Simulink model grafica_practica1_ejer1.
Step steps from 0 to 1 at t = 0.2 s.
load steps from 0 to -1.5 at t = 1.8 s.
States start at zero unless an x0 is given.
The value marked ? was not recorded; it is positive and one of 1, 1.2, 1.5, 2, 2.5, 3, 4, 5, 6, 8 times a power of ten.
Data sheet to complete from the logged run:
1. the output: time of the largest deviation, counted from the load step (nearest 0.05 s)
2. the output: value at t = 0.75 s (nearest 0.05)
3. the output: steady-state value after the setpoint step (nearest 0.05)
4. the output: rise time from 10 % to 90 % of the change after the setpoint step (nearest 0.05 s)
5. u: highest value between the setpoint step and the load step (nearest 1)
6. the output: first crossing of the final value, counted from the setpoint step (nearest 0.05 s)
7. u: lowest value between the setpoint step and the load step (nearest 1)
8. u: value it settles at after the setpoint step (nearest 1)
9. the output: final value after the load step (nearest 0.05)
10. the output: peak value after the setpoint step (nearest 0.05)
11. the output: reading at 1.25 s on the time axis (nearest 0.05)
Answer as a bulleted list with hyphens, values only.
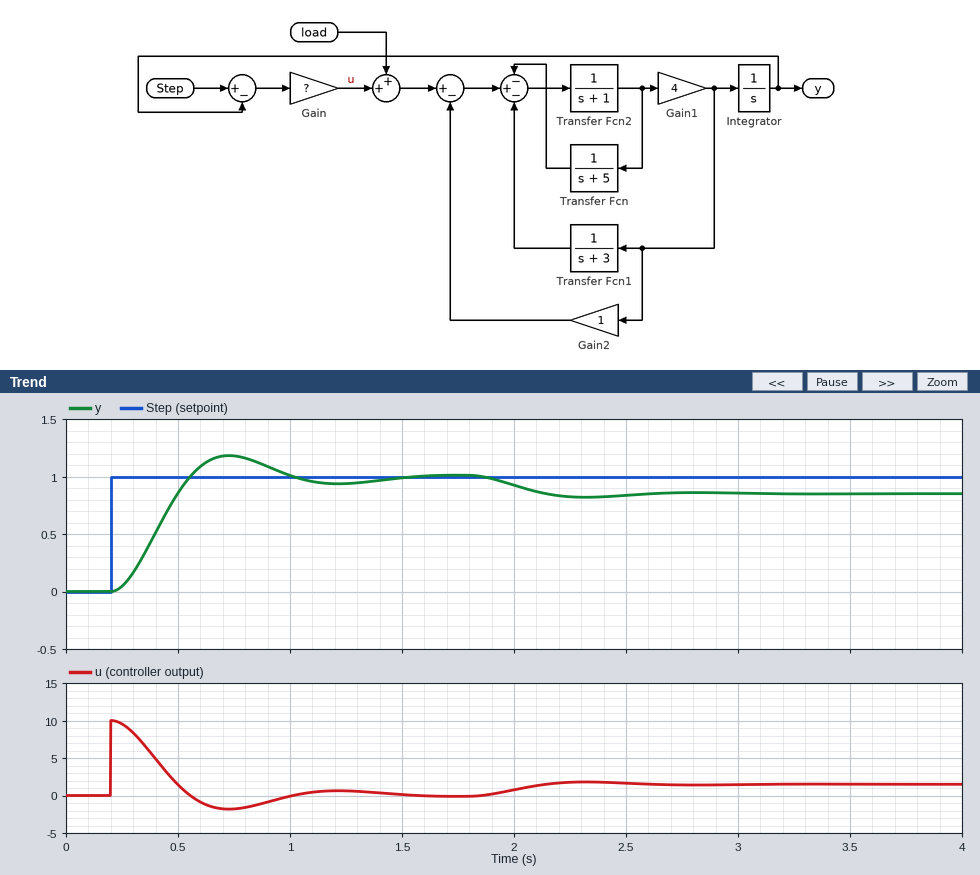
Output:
- 0.50 s
- 1.20
- 1.00
- 0.25 s
- 10
- 0.35 s
- -2
- 0
- 0.85
- 1.20
- 0.95
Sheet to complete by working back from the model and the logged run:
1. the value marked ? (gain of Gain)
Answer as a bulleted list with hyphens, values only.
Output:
- 10
